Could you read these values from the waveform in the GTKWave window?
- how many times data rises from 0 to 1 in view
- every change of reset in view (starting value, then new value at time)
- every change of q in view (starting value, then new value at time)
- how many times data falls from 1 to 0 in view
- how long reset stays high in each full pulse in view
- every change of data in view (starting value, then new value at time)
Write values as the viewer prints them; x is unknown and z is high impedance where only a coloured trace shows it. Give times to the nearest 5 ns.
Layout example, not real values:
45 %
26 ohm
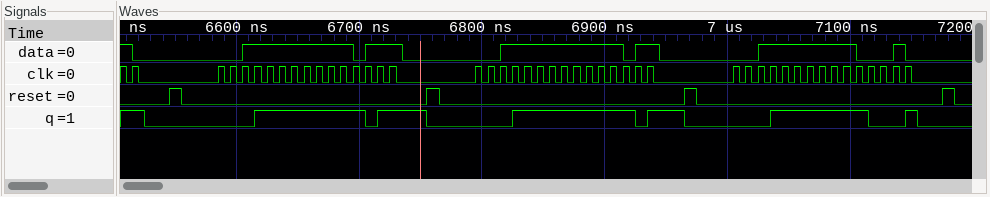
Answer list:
6
0, 1 at 6545 ns, 0 at 6555 ns, 1 at 6755 ns, 0 at 6765 ns, 1 at 6965 ns, 0 at 6975 ns, 1 at 7175 ns, 0 at 7185 ns
1, 0 at 6525 ns, 1 at 6615 ns, 0 at 6705 ns, 1 at 6715 ns, 0 at 6755 ns, 1 at 6825 ns, 0 at 6925 ns, 1 at 6935 ns, 0 at 6965 ns, 1 at 7035 ns, 0 at 7115 ns, 1 at 7145 ns, 0 at 7155 ns
7
10 ns, 10 ns, 10 ns, 10 ns
1, 0 at 6515 ns, 1 at 6605 ns, 0 at 6695 ns, 1 at 6705 ns, 0 at 6735 ns, 1 at 6815 ns, 0 at 6915 ns, 1 at 6925 ns, 0 at 6945 ns, 1 at 7025 ns, 0 at 7105 ns, 1 at 7135 ns, 0 at 7145 ns
